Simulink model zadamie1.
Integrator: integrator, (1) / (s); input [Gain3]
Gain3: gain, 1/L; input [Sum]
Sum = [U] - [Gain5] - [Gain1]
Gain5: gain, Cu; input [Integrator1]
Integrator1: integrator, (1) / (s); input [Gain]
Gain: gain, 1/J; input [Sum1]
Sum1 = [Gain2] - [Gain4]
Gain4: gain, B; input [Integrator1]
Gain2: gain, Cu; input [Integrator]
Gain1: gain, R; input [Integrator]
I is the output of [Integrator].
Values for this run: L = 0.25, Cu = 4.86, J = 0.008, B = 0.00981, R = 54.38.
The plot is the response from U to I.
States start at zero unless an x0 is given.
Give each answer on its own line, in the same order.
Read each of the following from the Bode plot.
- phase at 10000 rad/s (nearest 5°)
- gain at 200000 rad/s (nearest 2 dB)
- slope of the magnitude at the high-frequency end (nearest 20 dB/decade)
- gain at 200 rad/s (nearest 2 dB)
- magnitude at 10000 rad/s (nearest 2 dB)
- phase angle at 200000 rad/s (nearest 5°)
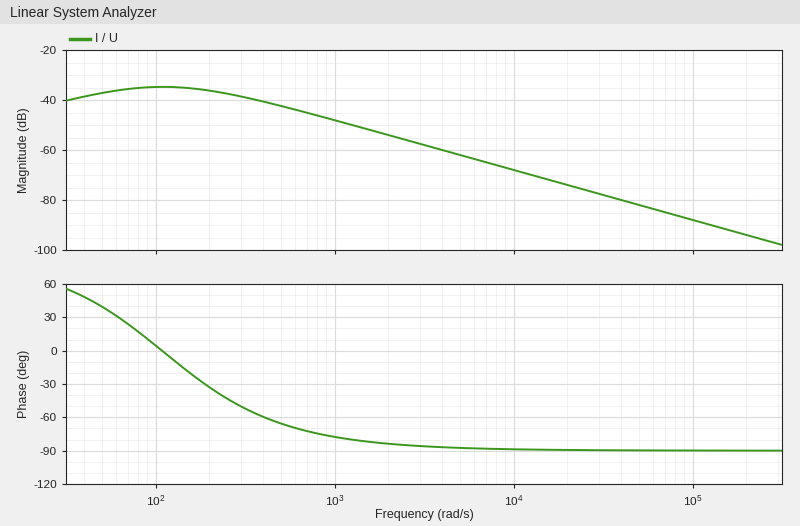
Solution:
-90°
-94 dB
-20 dB/decade
-36 dB
-68 dB
-90°
